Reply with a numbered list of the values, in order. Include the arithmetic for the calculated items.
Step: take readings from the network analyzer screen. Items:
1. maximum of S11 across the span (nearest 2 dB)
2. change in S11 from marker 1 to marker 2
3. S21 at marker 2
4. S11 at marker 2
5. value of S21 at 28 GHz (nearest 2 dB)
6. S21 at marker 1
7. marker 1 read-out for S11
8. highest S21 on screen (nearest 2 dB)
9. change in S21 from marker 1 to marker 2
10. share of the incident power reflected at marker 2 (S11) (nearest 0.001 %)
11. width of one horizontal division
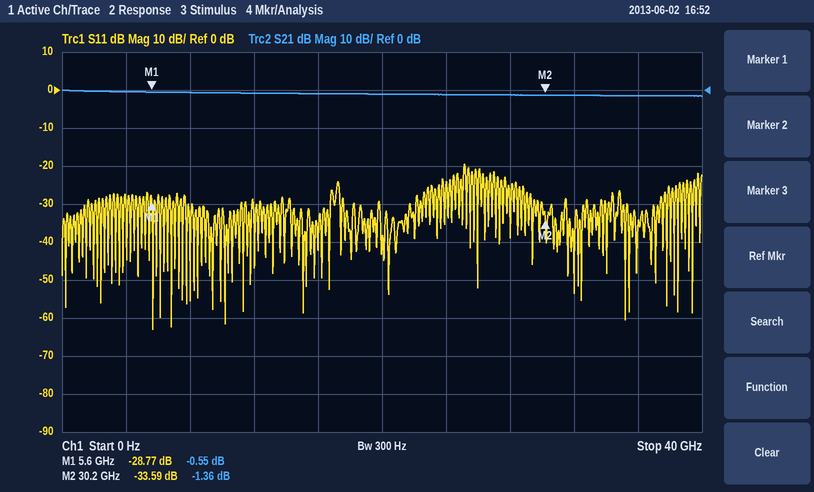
1. -20 dB
2. -33.59 − (-28.77) = -4.82 dB
3. -1.36 dB
4. -33.59 dB
5. -2 dB
6. -0.55 dB
7. -28.77 dB
8. 0 dB
9. -1.36 − (-0.55) = -0.81 dB
10. 10^(-33.59/10) ≈ 0.044 %
11. 4 GHz
